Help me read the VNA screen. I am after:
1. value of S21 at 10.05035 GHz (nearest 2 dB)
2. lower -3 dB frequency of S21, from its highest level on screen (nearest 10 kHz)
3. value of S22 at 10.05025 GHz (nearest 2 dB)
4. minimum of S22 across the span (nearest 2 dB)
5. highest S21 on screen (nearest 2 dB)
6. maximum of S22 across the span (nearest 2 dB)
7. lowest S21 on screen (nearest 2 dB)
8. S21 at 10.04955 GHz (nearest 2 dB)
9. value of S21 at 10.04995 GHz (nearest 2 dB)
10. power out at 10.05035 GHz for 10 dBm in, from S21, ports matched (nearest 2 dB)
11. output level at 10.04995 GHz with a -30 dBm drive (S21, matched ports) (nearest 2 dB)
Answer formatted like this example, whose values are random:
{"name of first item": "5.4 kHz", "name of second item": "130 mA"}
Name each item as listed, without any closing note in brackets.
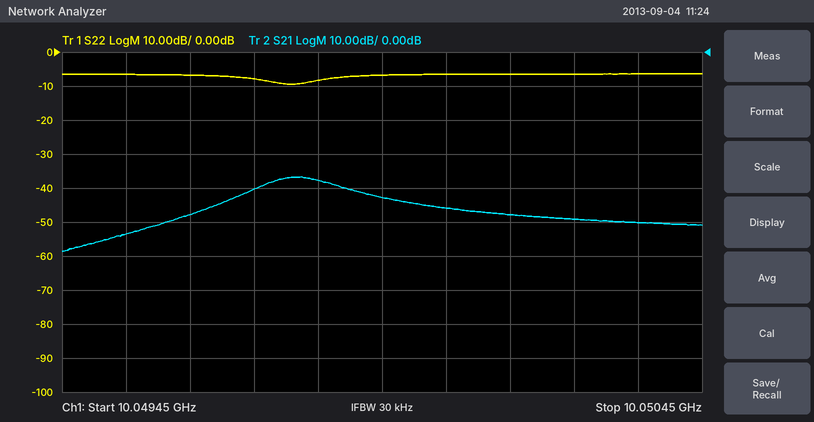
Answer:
{"value of S21 at 10.05035 GHz": "-50 dB", "lower -3 dB frequency of S21, from its highest level on screen": "10.04976 GHz", "value of S22 at 10.05025 GHz": "-6 dB", "minimum of S22 across the span": "-10 dB", "highest S21 on screen": "-36 dB", "maximum of S22 across the span": "-6 dB", "lowest S21 on screen": "-58 dB", "S21 at 10.04955 GHz": "-54 dB", "value of S21 at 10.04995 GHz": "-42 dB", "power out at 10.05035 GHz for 10 dBm in, from S21, ports matched": "-40 dBm", "output level at 10.04995 GHz with a -30 dBm drive (S21, matched ports)": "-72 dBm"}
